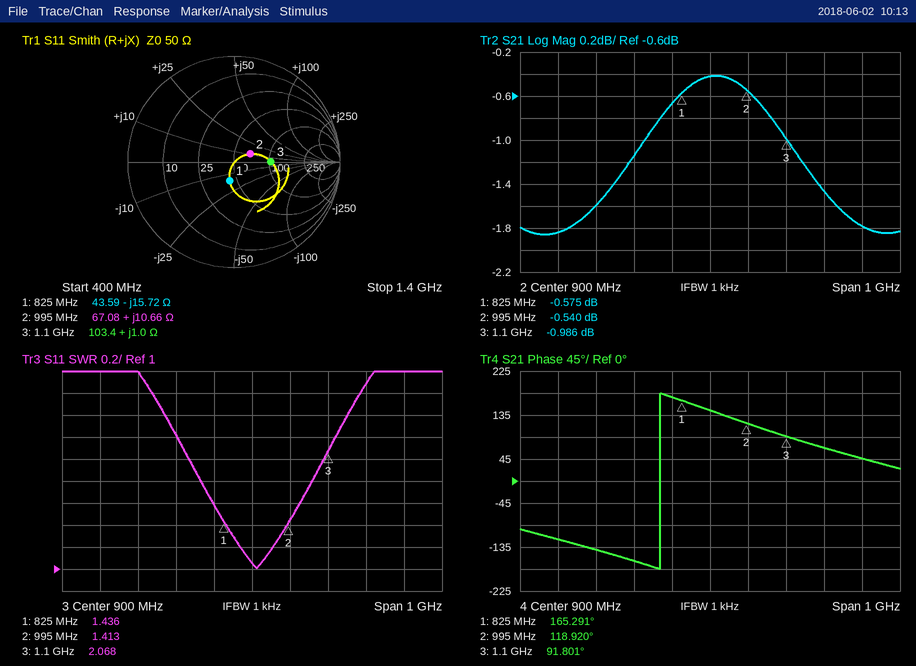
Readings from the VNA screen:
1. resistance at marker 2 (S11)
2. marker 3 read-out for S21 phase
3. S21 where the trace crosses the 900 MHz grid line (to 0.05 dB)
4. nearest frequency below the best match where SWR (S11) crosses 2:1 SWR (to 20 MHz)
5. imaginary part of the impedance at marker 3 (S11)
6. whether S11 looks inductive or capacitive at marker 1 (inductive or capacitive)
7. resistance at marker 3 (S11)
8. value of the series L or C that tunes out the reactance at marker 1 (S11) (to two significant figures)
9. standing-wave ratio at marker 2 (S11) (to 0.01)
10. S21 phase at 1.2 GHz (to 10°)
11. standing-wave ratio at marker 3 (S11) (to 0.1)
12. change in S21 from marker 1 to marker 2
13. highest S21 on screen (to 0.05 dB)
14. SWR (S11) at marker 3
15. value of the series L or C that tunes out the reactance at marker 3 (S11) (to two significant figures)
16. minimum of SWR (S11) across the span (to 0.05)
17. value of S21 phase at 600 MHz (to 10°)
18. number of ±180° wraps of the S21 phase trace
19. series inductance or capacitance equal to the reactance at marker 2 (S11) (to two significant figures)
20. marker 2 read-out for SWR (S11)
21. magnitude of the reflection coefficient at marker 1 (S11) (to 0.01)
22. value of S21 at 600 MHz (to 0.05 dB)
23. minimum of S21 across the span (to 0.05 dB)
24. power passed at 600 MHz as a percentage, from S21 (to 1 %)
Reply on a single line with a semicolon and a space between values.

67.08 Ω; 91.801°; -0.40 dB; 740 MHz; +1.0 Ω; capacitive; 103.4 Ω; 3.0 nH; 1.41; 70°; 2.1; 0.035 dB; -0.40 dB; 2.068; 140 pF; 1.00; -140°; 1; 1.7 nH; 1.413; 0.18; -1.60 dB; -1.85 dB; 69 %
